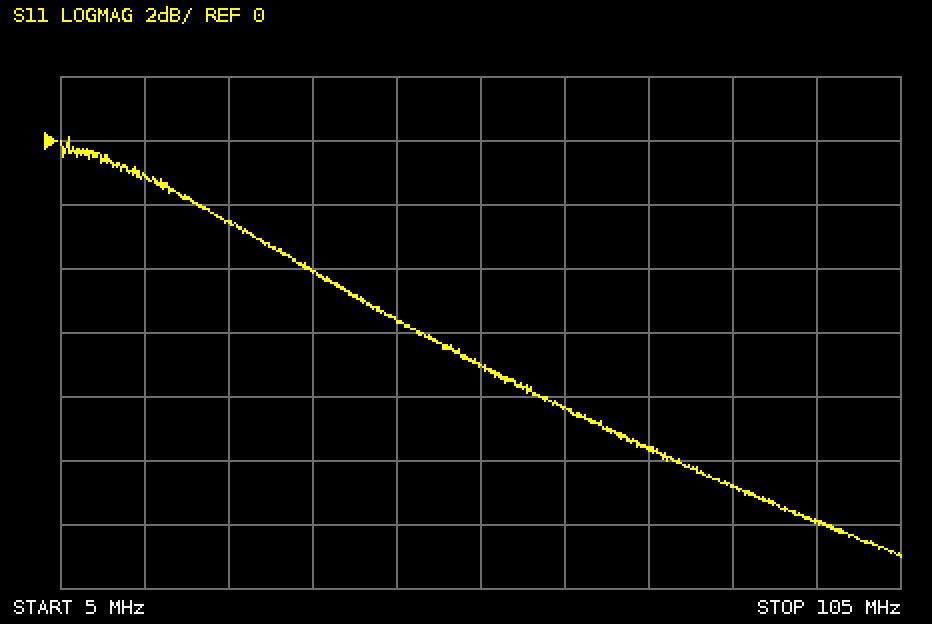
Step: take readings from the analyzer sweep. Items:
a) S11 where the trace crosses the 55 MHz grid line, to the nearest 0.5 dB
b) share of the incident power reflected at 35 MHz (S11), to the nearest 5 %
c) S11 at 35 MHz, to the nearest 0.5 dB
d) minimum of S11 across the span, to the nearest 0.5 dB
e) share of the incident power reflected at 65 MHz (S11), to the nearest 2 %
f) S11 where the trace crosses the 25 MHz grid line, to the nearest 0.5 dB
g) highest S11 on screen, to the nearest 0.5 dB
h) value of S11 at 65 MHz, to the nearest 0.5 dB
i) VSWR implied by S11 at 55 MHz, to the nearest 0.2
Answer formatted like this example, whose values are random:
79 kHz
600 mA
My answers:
-7.0 dB
40 %
-4.0 dB
-13.0 dB
14 %
-2.5 dB
0.0 dB
-8.5 dB
2.6
